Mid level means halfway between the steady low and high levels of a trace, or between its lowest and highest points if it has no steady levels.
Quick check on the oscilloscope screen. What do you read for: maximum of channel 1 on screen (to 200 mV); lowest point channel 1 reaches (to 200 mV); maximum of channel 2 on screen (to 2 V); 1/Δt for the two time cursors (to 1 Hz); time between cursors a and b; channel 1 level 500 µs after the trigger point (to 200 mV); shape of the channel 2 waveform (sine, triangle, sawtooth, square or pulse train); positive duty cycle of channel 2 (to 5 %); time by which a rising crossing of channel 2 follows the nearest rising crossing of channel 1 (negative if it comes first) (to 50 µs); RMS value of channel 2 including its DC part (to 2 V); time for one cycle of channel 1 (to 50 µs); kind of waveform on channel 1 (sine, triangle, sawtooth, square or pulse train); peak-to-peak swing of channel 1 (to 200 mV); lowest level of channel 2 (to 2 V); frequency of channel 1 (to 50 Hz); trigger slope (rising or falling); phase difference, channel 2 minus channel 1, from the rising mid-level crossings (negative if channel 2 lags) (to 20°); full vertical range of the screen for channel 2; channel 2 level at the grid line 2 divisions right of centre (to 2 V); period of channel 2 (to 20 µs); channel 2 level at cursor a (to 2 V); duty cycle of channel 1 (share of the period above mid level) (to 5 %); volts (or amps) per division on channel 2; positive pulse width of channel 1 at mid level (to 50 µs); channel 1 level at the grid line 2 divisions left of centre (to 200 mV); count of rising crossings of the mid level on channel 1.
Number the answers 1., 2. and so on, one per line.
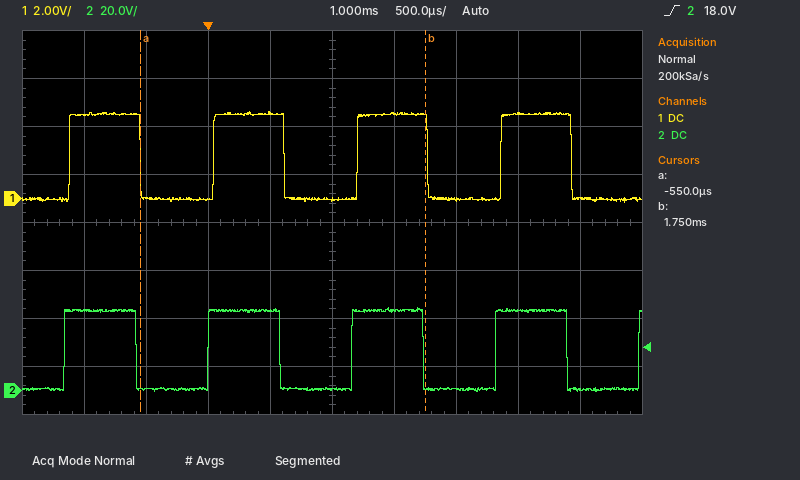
1. 3.6 V
2. -200 mV
3. 34 V
4. 435 Hz
5. 2.30 ms
6. 3.6 V
7. square
8. 50 %
9. -50 µs
10. 24 V
11. 1.15 ms
12. square
13. 3.8 V
14. 0 V
15. 850 Hz
16. rising
17. +20°
18. 160 V
19. 0 V
20. 1.16 ms
21. 0 V
22. 50 %
23. 20 V
24. 550 µs
25. 0.0 V
26. 4
